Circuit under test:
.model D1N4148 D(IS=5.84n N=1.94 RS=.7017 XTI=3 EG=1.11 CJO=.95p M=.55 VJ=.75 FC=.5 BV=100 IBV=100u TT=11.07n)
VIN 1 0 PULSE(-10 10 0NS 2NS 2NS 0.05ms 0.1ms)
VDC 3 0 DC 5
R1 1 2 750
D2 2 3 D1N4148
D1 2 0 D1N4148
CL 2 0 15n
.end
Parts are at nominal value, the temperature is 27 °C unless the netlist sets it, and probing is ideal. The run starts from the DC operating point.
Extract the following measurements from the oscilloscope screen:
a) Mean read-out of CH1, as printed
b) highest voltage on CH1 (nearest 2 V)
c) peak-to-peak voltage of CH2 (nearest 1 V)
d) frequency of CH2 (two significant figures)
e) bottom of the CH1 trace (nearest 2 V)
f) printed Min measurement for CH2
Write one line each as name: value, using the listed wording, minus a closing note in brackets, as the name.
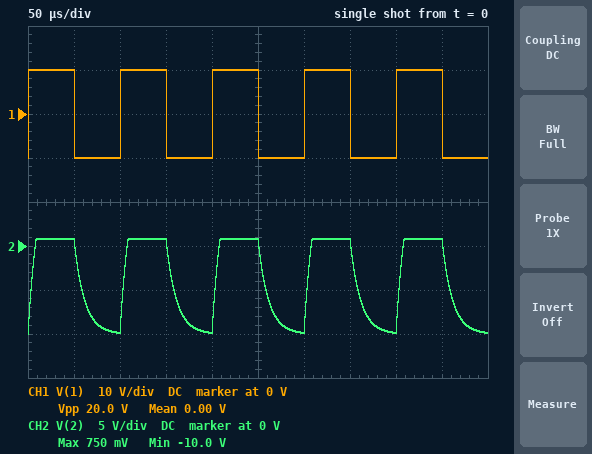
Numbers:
Mean read-out of CH1, as printed: 0.00 V
highest voltage on CH1: 10 V
peak-to-peak voltage of CH2: 11 V
frequency of CH2: 10 kHz
bottom of the CH1 trace: -10 V
printed Min measurement for CH2: -10.0 V
